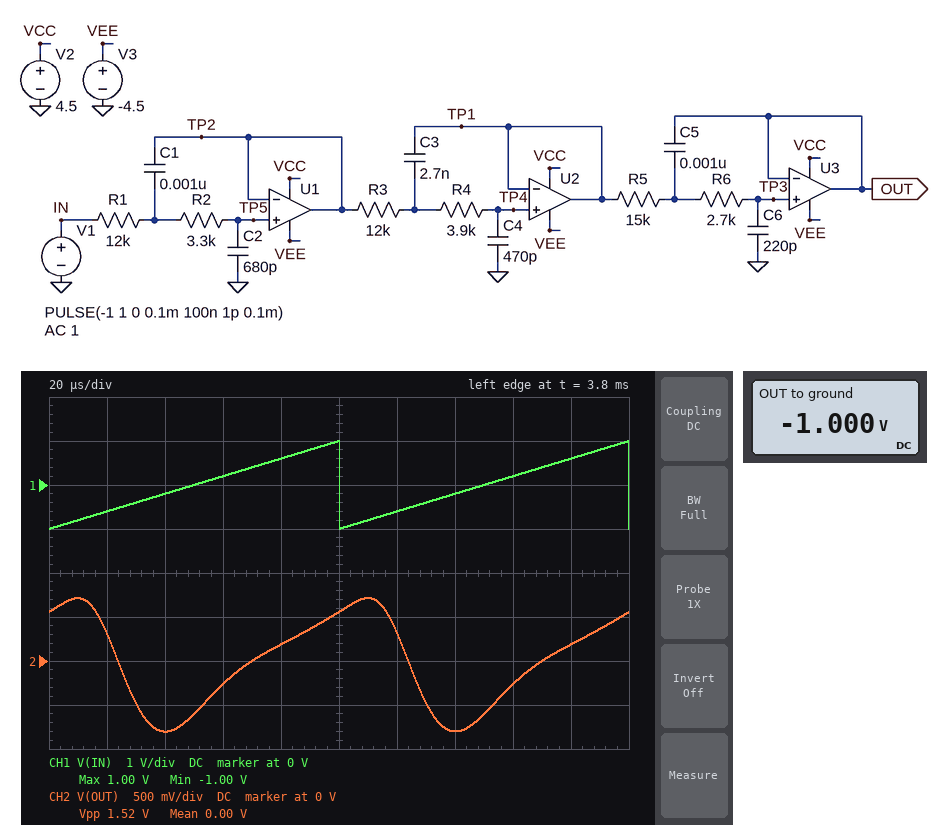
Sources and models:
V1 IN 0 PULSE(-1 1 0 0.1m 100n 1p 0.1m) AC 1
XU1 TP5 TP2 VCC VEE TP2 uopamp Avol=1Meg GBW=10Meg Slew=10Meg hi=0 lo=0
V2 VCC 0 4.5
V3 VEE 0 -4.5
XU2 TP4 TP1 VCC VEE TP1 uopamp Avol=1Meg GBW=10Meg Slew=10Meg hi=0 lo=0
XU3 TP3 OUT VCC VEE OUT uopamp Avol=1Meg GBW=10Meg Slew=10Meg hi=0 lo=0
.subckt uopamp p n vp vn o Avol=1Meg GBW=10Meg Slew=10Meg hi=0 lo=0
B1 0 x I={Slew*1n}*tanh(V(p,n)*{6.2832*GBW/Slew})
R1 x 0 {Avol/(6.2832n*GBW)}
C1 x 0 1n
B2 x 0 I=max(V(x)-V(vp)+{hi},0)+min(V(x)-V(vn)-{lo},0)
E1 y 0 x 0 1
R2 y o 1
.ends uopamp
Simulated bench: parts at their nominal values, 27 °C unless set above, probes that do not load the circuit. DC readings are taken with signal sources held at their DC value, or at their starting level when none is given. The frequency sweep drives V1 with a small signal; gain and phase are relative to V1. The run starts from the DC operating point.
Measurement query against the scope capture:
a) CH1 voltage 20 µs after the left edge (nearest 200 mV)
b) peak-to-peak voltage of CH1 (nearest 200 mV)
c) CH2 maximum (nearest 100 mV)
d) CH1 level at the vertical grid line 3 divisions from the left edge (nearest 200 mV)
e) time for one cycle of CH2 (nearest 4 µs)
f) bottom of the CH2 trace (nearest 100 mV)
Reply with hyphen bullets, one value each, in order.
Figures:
- -600 mV
- 2.0 V
- 700 mV
- 200 mV
- 100 µs
- -800 mV
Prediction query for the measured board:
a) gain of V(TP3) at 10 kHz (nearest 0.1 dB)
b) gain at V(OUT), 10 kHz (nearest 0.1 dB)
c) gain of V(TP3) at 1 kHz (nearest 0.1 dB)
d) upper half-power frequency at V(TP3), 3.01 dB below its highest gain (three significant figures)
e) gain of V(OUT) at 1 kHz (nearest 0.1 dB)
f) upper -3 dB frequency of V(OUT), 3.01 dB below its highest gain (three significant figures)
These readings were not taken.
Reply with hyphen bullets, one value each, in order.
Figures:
- 0.1 dB
- 0.1 dB
- 0 dB
- 20.7 kHz
- 0 dB
- 20.7 kHz
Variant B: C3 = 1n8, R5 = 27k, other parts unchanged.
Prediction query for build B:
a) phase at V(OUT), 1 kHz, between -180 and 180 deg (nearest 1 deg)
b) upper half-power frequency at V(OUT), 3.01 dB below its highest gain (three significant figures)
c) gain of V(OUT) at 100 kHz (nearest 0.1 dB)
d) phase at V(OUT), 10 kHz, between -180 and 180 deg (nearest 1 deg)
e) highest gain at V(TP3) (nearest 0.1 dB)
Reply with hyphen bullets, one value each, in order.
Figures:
- -9 deg
- 17.9 kHz
- -61.9 dB
- -89 deg
- 0 dB
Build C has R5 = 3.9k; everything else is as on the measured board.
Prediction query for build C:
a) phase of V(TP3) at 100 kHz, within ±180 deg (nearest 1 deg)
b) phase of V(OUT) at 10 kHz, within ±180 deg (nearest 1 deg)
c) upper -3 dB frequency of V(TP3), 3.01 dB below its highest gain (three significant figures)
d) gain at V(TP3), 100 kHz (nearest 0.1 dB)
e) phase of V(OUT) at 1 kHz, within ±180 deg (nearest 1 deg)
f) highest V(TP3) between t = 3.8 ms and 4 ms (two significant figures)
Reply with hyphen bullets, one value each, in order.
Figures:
- -42 deg
- -73 deg
- 20.8 kHz
- -47.9 dB
- -7 deg
- 730 mV
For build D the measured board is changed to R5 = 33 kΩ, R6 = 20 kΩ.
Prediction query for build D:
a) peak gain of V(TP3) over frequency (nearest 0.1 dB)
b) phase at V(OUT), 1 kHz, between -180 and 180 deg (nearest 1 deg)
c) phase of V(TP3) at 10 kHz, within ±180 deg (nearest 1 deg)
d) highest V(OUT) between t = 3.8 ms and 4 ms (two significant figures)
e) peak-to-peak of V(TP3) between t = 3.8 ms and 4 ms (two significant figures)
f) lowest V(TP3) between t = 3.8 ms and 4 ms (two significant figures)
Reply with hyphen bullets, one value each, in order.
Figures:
- 1.5 dB
- -11 deg
- -128 deg
- 730 mV
- 1.6 V
- -830 mV
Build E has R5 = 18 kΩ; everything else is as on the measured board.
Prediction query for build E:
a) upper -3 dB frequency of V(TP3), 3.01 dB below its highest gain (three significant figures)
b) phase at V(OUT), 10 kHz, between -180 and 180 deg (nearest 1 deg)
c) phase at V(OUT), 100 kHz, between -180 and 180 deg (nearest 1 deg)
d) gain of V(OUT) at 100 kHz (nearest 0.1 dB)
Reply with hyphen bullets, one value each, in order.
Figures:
- 20.5 kHz
- -85 deg
- -95 deg
- -61.5 dB
